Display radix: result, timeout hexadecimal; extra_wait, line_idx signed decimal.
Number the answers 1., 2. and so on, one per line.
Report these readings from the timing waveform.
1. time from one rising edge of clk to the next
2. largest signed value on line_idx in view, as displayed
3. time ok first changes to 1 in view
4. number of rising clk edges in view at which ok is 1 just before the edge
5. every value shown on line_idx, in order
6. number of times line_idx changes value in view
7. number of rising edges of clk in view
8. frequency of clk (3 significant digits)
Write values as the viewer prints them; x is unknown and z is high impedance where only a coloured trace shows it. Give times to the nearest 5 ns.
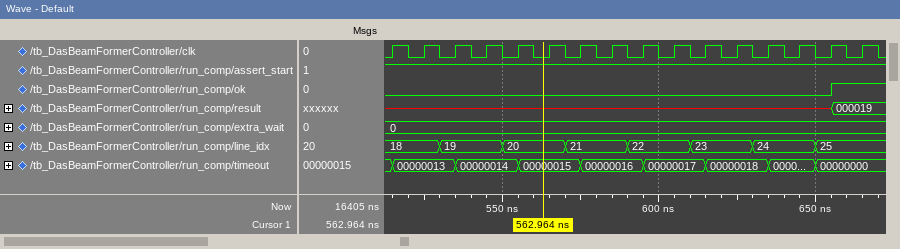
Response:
1. 10 ns
2. 25
3. 655 ns
4. 1
5. 18, 19, 20, 21, 22, 23, 24, 25
6. 7
7. 16
8. 100 MHz
